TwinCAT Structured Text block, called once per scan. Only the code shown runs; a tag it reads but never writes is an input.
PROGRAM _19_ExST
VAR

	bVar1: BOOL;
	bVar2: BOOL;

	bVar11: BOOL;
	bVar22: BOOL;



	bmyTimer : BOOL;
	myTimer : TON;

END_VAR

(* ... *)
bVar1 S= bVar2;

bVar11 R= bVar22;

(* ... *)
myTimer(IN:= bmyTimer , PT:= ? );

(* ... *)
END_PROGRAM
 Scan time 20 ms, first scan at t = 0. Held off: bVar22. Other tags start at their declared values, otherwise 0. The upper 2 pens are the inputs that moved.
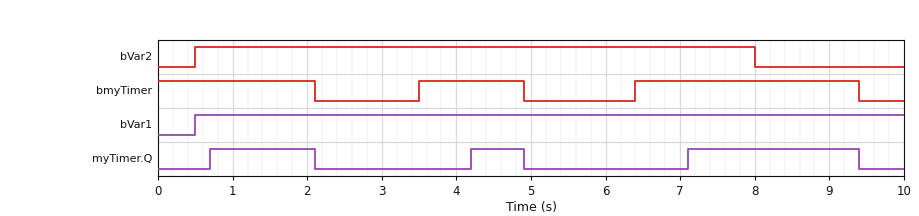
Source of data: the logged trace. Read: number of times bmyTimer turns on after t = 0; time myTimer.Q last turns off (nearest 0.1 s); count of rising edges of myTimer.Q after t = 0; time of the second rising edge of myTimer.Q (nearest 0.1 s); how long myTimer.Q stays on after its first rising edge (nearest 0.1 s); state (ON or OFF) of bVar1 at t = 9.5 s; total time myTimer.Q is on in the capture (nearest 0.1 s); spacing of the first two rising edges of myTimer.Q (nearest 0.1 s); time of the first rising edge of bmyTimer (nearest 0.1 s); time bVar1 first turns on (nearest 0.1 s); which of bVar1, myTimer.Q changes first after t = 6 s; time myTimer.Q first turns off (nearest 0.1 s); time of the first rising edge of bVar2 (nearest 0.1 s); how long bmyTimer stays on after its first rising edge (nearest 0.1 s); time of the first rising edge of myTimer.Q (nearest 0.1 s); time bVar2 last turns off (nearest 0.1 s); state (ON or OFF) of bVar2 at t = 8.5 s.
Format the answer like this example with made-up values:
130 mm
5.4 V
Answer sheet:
2
9.4 s
3
4.2 s
1.4 s
ON
4.4 s
3.5 s
3.5 s
0.5 s
myTimer.Q
2.1 s
0.5 s
1.4 s
0.7 s
8.0 s
OFF
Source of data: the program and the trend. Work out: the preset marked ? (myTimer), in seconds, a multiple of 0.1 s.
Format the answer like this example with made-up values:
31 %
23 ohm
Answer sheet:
0.7 s
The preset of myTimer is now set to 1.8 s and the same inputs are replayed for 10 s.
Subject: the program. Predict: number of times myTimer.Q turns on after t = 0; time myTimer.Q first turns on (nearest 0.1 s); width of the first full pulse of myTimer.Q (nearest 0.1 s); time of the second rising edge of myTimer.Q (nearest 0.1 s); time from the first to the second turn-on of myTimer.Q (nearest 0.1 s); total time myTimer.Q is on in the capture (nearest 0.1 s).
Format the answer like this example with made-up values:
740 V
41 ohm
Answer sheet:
2
1.8 s
0.3 s
8.2 s
6.4 s
1.5 s
